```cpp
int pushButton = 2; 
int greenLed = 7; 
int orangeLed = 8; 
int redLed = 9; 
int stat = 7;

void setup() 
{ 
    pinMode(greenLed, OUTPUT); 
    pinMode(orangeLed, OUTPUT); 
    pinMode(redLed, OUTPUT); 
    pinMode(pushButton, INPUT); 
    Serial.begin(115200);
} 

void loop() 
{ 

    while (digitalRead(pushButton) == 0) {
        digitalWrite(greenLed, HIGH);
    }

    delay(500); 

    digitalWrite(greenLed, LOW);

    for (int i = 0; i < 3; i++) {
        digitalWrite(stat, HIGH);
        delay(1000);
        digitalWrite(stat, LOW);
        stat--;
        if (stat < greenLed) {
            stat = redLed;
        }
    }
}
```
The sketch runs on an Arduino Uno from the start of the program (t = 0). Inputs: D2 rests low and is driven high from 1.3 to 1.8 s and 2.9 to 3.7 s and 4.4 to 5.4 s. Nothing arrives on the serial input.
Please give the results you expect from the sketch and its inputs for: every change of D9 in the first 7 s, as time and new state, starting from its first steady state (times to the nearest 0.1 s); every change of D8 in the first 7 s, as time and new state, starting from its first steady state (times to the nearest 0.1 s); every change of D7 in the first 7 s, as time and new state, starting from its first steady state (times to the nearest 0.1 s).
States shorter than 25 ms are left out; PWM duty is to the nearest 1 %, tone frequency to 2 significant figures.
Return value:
0 s low; 2.8 s high; 3.8 s low; 6.3 s high
0 s low; 3.8 s high; 4.8 s low
0 s high; 2.8 s low; 5.3 s high; 6.3 s low
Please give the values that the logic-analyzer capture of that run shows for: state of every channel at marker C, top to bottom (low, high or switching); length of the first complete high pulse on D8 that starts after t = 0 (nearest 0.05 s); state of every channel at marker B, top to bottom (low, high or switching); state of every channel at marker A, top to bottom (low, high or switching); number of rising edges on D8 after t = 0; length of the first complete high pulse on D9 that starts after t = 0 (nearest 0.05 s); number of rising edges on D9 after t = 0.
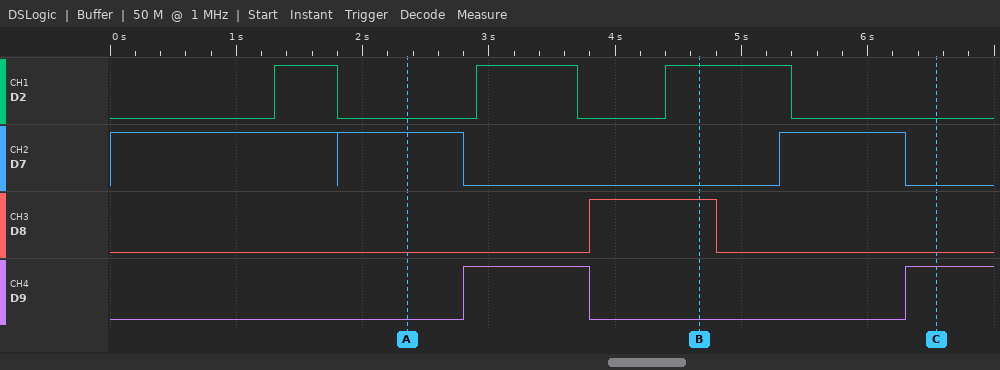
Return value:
D2 low, D7 low, D8 low, D9 high
1.00 s
D2 high, D7 low, D8 high, D9 low
D2 low, D7 high, D8 low, D9 low
1
1.00 s
2
